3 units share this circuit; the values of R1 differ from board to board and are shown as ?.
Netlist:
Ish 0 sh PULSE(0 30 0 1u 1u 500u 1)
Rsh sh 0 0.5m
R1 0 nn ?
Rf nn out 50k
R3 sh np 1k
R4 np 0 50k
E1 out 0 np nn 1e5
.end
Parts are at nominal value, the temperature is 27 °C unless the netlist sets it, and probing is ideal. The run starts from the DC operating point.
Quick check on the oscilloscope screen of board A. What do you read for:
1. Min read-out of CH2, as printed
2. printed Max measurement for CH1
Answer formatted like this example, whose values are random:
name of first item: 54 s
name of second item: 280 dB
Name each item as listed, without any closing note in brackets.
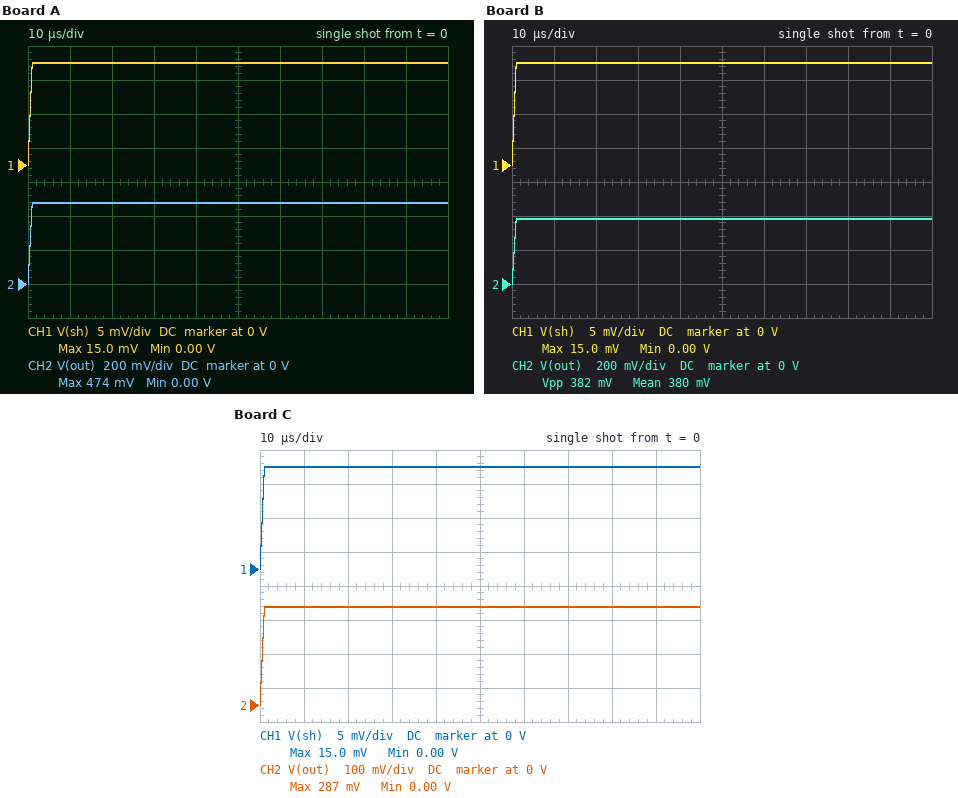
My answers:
Min read-out of CH2, as printed: 0.00 V
printed Max measurement for CH1: 15.0 mV
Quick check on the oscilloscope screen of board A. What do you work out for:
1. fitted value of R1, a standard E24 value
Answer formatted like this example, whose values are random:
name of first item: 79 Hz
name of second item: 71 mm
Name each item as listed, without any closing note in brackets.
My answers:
fitted value of R1, a standard E24 value: 1.6 kΩ
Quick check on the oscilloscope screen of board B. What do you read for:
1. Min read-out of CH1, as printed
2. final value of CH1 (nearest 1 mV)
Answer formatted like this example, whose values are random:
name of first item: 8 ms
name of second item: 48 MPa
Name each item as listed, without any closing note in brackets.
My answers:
Min read-out of CH1, as printed: 0.00 V
final value of CH1: 15 mV
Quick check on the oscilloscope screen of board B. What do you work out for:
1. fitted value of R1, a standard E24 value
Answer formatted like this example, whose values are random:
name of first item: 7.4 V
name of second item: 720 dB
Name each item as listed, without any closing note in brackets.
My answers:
fitted value of R1, a standard E24 value: 2 kΩ
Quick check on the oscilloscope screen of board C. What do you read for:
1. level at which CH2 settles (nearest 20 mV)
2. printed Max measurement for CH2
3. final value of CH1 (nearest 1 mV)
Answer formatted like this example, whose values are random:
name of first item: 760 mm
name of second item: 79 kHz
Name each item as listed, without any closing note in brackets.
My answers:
level at which CH2 settles: 280 mV
printed Max measurement for CH2: 287 mV
final value of CH1: 15 mV
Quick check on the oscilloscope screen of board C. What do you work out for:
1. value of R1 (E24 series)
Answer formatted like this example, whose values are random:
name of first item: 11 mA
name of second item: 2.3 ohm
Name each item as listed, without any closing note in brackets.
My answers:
value of R1: 2.7 kΩ
